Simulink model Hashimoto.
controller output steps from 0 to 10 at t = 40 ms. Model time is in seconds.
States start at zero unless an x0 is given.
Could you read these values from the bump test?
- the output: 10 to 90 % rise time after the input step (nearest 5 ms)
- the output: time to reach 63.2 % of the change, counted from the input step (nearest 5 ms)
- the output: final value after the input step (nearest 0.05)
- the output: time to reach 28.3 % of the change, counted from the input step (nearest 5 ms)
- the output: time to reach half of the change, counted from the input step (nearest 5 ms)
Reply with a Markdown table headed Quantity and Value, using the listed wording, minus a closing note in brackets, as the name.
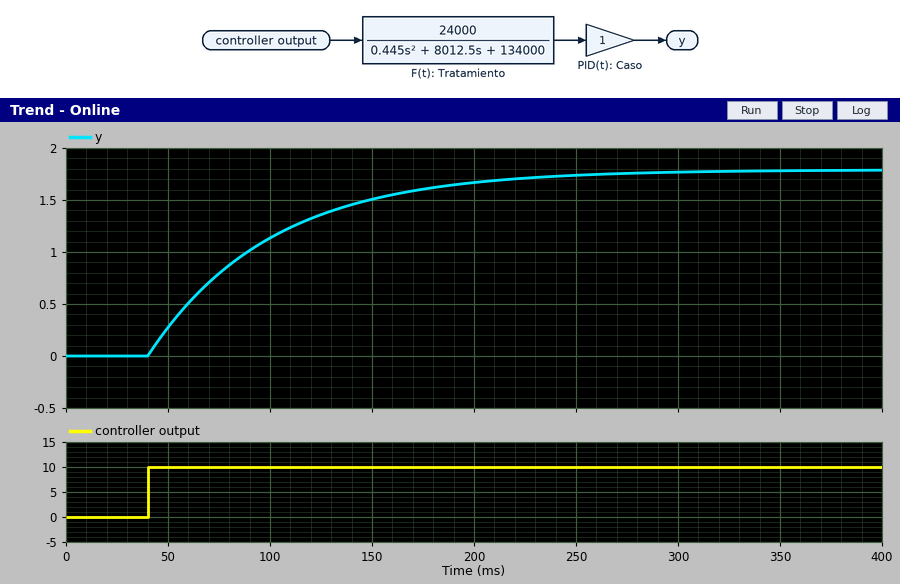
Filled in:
| Quantity | Value |
|---|---|
| the output: 10 to 90 % rise time after the input step | 130 ms |
| the output: time to reach 63.2 % of the change, counted from the input step | 60 ms |
| the output: final value after the input step | 1.80 |
| the output: time to reach 28.3 % of the change, counted from the input step | 20 ms |
| the output: time to reach half of the change, counted from the input step | 40 ms |
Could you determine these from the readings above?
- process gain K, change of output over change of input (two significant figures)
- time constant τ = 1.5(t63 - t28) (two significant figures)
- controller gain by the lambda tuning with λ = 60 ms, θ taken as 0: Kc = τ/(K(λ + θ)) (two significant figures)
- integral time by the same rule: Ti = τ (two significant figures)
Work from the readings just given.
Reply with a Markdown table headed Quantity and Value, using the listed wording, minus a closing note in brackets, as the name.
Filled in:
| Quantity | Value |
|---|---|
| process gain K, change of output over change of input | 0.18 |
| time constant τ = 1.5(t63 - t28) | 60 ms |
| controller gain by the lambda tuning with λ = 60 ms, θ taken as 0: Kc = τ/(K(λ + θ)) | 5.6 |
| integral time by the same rule: Ti = τ | 60 ms |
